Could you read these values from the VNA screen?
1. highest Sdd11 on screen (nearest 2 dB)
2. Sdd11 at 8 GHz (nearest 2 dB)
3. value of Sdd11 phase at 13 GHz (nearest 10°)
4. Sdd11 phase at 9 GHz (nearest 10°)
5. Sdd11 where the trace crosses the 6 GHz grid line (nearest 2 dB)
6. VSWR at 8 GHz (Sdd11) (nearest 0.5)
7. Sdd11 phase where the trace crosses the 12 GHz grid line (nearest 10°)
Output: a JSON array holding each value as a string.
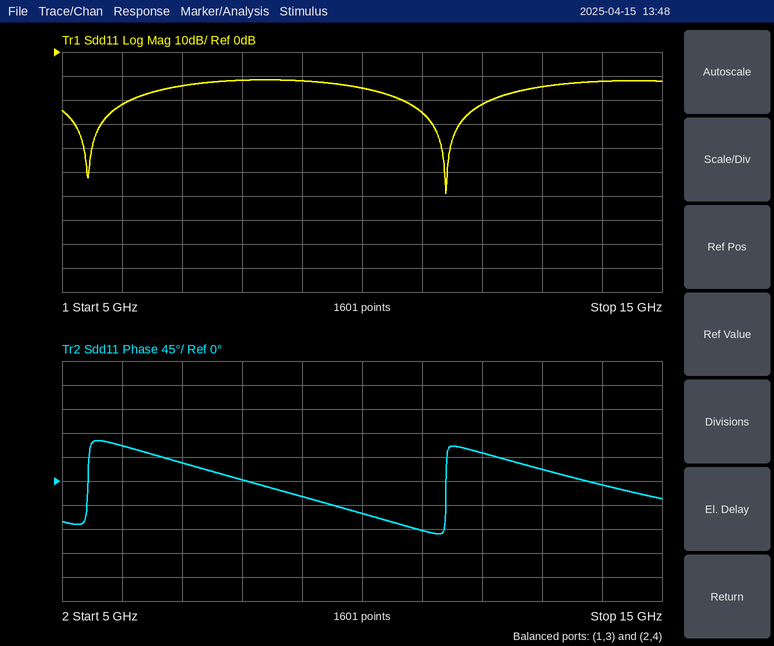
["-12 dB", "-12 dB", "20°", "-30°", "-22 dB", "1.5", "50°"]
